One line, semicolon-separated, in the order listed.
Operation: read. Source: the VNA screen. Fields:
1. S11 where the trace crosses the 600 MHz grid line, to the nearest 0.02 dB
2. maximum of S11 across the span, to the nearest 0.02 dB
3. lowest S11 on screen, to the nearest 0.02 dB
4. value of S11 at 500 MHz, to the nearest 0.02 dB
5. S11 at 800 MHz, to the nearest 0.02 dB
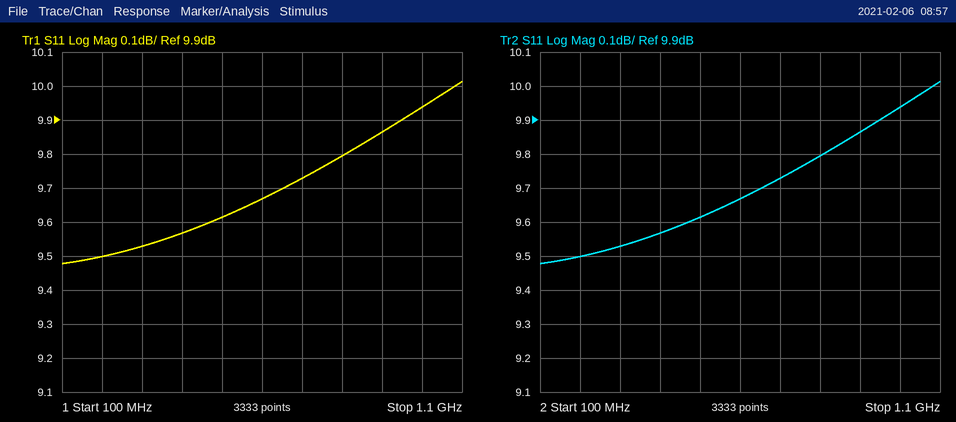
9.66 dB; 10.02 dB; 9.48 dB; 9.62 dB; 9.80 dB
